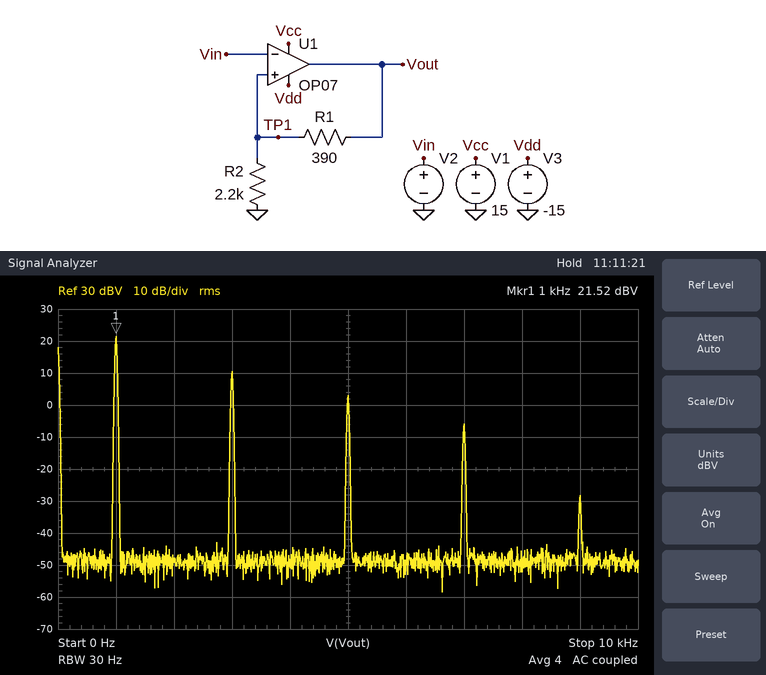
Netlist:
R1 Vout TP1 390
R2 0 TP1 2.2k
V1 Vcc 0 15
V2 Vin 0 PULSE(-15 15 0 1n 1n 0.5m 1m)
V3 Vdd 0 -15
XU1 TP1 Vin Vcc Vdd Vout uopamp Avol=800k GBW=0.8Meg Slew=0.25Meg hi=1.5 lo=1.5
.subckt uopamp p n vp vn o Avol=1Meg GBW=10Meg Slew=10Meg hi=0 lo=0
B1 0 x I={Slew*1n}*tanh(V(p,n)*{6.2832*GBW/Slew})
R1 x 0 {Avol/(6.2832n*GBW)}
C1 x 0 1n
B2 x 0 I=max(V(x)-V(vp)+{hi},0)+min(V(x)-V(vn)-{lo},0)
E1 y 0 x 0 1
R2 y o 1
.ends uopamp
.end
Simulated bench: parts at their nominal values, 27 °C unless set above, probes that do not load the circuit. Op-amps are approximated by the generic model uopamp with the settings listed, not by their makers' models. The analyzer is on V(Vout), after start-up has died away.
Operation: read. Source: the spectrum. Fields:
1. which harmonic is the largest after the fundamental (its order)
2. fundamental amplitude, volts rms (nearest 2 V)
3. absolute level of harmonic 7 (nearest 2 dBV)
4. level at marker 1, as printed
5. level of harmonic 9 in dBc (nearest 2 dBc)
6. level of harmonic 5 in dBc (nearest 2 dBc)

3
12 V
-6 dBV
21.52 dBV
-50 dBc
-18 dBc
